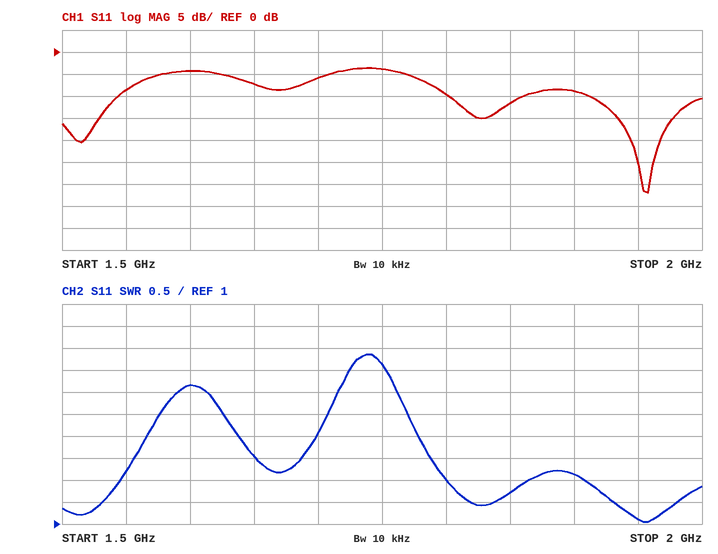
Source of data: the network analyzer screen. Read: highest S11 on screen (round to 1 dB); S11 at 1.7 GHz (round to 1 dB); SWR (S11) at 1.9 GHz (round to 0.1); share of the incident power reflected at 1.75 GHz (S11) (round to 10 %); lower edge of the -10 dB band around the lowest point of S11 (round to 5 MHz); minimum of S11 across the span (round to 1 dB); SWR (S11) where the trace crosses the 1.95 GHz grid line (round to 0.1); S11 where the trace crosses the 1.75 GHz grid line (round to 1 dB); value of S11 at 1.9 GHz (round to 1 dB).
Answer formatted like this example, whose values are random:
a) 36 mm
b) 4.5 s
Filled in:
a) -4 dB
b) -6 dB
c) 2.1
d) 40 %
e) 1.910 GHz
f) -32 dB
g) 1.1
h) -4 dB
i) -9 dB
